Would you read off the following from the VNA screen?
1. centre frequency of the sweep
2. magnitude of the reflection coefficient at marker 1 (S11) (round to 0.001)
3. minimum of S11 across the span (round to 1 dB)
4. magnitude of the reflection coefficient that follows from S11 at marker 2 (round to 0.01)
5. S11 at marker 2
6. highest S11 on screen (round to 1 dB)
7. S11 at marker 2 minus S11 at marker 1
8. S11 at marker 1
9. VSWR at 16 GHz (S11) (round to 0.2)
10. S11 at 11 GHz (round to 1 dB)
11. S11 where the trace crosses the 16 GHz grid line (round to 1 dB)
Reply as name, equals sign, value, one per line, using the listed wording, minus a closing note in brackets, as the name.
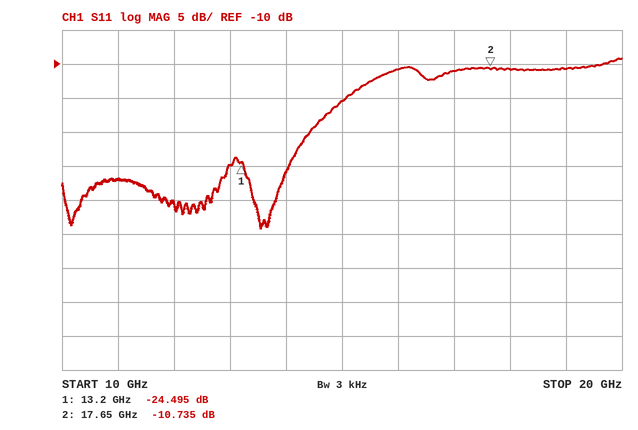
centre frequency of the sweep = 15 GHz
magnitude of the reflection coefficient at marker 1 (S11) = 0.060
minimum of S11 across the span = -34 dB
magnitude of the reflection coefficient that follows from S11 at marker 2 = 0.29
S11 at marker 2 = -10.735 dB
highest S11 on screen = -9 dB
S11 at marker 2 minus S11 at marker 1 = 13.760 dB
S11 at marker 1 = -24.495 dB
VSWR at 16 GHz (S11) = 1.8
S11 at 11 GHz = -27 dB
S11 where the trace crosses the 16 GHz grid line = -11 dB
